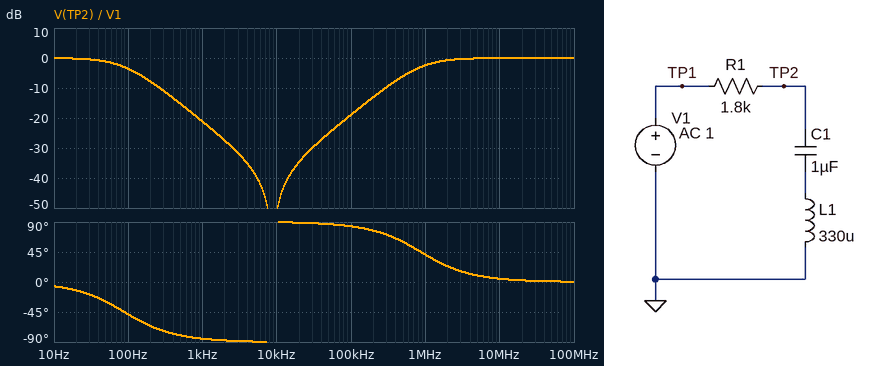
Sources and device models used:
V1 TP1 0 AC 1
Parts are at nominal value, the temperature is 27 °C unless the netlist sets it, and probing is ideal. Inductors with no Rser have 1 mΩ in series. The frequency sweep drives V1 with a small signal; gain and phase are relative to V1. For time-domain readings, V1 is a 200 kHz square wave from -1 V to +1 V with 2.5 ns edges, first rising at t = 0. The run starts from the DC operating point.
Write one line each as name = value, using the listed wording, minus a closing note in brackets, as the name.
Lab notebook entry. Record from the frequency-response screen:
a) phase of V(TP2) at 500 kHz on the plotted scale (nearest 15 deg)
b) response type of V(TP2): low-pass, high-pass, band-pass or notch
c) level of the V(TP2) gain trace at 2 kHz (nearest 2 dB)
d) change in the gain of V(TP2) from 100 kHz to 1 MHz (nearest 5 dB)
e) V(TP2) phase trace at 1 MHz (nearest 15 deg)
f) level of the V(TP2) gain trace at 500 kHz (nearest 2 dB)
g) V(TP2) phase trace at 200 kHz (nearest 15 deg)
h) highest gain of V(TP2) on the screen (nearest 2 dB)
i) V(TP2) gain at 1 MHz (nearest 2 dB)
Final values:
phase of V(TP2) at 500 kHz on the plotted scale = 60 deg
response type of V(TP2): low-pass, high-pass, band-pass or notch = notch
level of the V(TP2) gain trace at 2 kHz = -28 dB
change in the gain of V(TP2) from 100 kHz to 1 MHz = 15 dB
V(TP2) phase trace at 1 MHz = 45 deg
level of the V(TP2) gain trace at 500 kHz = -6 dB
V(TP2) phase trace at 200 kHz = 75 deg
highest gain of V(TP2) on the screen = 0 dB
V(TP2) gain at 1 MHz = -2 dB
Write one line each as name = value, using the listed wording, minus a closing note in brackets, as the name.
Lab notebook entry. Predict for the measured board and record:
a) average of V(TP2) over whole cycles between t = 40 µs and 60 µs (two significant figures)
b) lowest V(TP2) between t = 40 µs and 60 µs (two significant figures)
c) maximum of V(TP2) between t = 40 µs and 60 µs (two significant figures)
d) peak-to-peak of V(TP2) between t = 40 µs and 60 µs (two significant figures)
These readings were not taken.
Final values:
average of V(TP2) over whole cycles between t = 40 µs and 60 µs = -970 mV
lowest V(TP2) between t = 40 µs and 60 µs = -3.0 V
maximum of V(TP2) between t = 40 µs and 60 µs = 1.0 V
peak-to-peak of V(TP2) between t = 40 µs and 60 µs = 4.0 V
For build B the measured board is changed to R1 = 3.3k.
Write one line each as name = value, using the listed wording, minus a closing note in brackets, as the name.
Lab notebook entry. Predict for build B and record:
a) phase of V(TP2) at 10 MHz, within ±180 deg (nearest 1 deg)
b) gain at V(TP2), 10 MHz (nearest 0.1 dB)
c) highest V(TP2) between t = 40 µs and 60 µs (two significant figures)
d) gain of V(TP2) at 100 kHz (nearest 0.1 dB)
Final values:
phase of V(TP2) at 10 MHz, within ±180 deg = 9 deg
gain at V(TP2), 10 MHz = -0.1 dB
highest V(TP2) between t = 40 µs and 60 µs = 990 mV
gain of V(TP2) at 100 kHz = -24.1 dB
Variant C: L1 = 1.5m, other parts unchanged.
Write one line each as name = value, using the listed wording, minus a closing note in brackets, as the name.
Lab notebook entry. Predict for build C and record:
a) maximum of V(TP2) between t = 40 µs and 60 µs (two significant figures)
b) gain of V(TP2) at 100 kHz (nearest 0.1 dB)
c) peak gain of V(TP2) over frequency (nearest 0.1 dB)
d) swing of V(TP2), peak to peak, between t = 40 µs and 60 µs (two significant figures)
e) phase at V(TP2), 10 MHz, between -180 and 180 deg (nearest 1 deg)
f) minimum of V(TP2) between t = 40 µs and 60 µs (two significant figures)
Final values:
maximum of V(TP2) between t = 40 µs and 60 µs = 930 mV
gain of V(TP2) at 100 kHz = -6.7 dB
peak gain of V(TP2) over frequency = 0 dB
swing of V(TP2), peak to peak, between t = 40 µs and 60 µs = 3.8 V
phase at V(TP2), 10 MHz, between -180 and 180 deg = 1 deg
minimum of V(TP2) between t = 40 µs and 60 µs = -2.9 V
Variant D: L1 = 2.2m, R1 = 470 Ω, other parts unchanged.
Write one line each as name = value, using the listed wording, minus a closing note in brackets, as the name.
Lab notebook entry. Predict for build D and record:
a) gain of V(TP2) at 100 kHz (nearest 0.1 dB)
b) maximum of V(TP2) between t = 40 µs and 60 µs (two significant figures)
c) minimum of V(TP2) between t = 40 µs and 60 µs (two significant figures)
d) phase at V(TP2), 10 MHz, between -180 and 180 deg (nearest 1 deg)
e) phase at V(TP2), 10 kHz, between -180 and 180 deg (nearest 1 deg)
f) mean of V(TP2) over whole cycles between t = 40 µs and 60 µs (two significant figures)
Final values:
gain of V(TP2) at 100 kHz = -0.5 dB
maximum of V(TP2) between t = 40 µs and 60 µs = 360 mV
minimum of V(TP2) between t = 40 µs and 60 µs = -2.2 V
phase at V(TP2), 10 MHz, between -180 and 180 deg = 0 deg
phase at V(TP2), 10 kHz, between -180 and 180 deg = 75 deg
mean of V(TP2) over whole cycles between t = 40 µs and 60 µs = -910 mV
